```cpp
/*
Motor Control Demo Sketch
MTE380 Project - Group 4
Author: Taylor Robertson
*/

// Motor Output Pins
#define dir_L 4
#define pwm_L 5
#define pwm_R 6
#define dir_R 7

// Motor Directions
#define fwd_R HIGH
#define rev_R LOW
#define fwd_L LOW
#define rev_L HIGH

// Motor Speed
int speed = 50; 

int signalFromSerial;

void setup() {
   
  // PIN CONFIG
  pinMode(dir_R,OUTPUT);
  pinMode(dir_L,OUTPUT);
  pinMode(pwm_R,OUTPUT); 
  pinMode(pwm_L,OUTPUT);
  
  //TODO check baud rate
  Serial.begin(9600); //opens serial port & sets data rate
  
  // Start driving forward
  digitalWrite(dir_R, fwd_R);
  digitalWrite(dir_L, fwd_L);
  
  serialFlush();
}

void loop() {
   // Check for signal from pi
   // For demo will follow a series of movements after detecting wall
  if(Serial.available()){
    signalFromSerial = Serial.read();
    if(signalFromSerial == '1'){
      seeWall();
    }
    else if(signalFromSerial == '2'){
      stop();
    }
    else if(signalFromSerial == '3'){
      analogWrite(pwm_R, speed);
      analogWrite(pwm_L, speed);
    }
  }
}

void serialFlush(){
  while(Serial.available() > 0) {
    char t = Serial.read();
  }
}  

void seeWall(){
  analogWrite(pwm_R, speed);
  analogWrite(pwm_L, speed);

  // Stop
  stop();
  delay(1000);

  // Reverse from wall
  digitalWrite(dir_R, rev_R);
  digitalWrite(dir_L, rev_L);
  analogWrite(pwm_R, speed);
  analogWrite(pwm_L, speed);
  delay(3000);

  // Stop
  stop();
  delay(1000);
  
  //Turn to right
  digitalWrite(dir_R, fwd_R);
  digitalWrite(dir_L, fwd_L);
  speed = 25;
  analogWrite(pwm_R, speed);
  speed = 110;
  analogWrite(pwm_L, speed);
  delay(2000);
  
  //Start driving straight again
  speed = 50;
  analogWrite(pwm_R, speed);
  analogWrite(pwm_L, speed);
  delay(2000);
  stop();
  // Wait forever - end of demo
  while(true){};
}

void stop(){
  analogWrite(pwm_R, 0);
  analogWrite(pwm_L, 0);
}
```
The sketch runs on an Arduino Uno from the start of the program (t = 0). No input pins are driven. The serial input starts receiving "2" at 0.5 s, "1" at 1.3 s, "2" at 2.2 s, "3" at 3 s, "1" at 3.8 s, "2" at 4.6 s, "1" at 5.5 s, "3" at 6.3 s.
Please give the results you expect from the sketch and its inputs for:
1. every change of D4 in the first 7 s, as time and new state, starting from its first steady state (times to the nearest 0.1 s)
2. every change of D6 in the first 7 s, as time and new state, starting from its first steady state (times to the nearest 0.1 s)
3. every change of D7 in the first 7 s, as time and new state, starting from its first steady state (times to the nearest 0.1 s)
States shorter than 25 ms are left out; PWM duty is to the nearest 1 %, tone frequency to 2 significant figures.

0 s low; 2.3 s high; 6.3 s low
0 s low; 2.3 s PWM 20 %; 5.3 s low; 6.3 s PWM 10 %
0 s high; 2.3 s low; 6.3 s high
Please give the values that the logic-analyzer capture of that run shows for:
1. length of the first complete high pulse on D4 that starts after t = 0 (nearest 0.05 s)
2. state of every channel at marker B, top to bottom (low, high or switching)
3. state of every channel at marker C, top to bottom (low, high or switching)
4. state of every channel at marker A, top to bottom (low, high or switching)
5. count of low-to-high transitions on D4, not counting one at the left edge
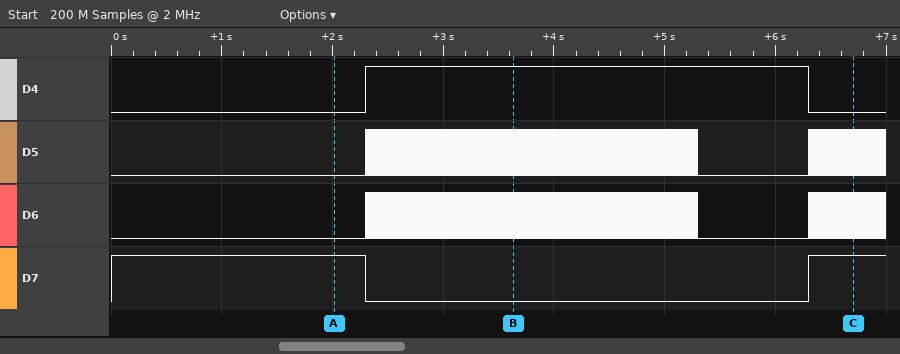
4.00 s
D4 high, D5 switching, D6 switching, D7 low
D4 low, D5 switching, D6 switching, D7 high
D4 low, D5 low, D6 low, D7 high
1
